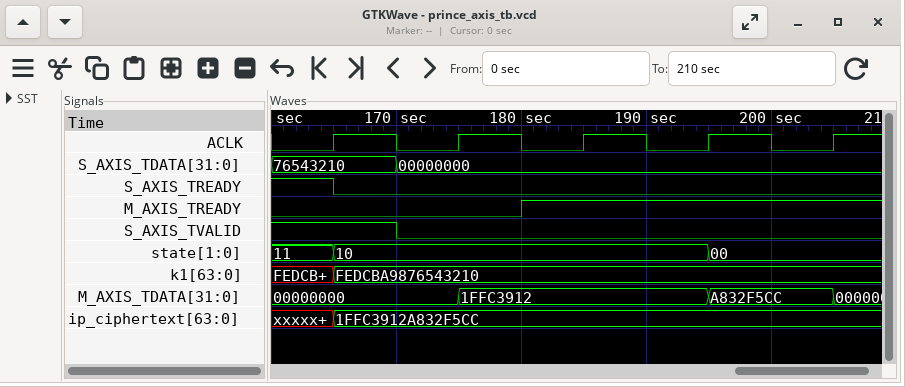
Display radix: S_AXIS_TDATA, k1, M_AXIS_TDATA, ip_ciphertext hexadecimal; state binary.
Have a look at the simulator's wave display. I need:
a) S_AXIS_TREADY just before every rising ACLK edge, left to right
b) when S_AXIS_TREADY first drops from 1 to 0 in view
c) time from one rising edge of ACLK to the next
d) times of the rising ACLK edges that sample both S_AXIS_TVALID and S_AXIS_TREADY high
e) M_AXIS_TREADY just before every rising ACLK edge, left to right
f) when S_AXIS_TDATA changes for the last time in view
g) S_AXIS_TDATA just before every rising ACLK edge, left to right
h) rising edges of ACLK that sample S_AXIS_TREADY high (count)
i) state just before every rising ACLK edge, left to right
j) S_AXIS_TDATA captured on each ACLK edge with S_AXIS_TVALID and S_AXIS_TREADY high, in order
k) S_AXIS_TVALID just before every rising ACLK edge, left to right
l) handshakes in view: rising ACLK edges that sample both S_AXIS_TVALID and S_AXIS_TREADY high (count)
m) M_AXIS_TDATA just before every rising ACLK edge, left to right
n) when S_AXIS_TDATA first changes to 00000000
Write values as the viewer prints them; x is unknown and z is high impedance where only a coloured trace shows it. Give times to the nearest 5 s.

1 0 0 0 0
165 s
10 s
165 s
0 0 1 1 1
170 s
76543210, 00000000, 00000000, 00000000, 00000000
1
11, 10, 10, 10, 00
76543210
1 0 0 0 0
1
00000000, 00000000, 1FFC3912, 1FFC3912, A832F5CC
170 s
